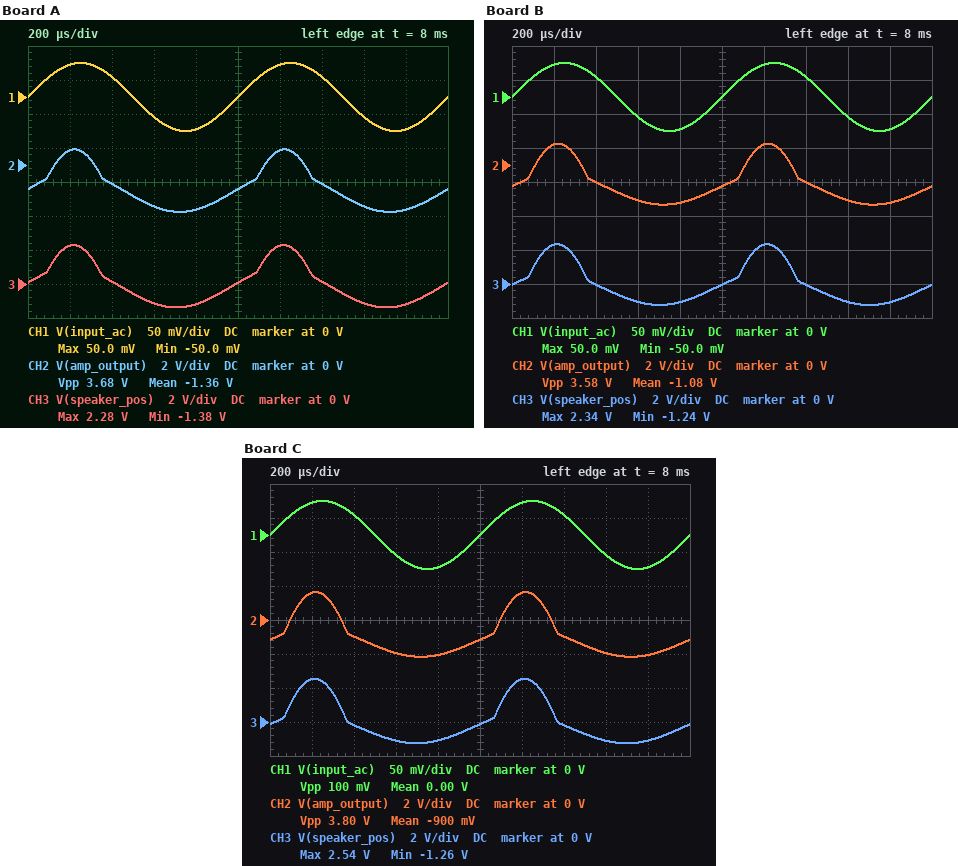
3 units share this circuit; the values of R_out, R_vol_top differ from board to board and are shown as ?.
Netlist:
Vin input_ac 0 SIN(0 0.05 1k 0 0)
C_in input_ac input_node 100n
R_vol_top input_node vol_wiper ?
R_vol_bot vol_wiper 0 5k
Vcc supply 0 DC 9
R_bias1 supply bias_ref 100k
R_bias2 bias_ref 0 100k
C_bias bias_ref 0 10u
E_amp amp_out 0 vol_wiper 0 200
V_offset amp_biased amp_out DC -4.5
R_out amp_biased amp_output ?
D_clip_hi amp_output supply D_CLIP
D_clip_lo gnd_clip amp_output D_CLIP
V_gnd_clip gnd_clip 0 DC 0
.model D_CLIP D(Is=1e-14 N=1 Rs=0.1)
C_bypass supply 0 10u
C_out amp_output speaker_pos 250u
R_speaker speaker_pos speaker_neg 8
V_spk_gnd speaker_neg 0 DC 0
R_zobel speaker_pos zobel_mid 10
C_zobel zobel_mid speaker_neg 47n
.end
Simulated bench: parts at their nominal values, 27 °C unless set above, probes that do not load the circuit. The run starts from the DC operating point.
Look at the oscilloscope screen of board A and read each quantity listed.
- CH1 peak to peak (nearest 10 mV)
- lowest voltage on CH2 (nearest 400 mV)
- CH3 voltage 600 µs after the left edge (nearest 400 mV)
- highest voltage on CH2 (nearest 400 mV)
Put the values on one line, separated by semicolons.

100 mV; -2.8 V; -1.2 V; 800 mV
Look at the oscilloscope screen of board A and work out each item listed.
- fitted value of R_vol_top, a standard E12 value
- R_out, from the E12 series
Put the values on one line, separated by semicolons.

3.9 kΩ; 0.39 Ω
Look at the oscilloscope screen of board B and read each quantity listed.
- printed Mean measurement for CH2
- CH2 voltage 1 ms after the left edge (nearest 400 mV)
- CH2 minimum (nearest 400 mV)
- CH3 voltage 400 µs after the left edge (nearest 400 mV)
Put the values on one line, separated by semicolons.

-1.08 V; -1.2 V; -2.4 V; 0 V
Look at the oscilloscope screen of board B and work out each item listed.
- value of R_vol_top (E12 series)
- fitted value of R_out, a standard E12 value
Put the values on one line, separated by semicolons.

3.3 kΩ; 0.56 Ω
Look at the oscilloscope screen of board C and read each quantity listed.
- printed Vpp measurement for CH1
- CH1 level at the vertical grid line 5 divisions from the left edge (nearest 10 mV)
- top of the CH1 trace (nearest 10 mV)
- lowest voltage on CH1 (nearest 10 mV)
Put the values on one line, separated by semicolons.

100 mV; 0 V; 50 mV; -50 mV
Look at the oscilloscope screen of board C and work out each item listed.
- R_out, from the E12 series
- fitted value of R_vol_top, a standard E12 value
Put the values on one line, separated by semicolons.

0.68 Ω; 2.7 kΩ
